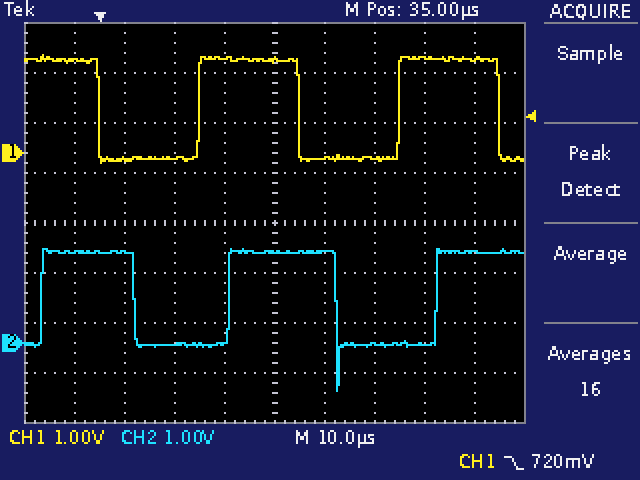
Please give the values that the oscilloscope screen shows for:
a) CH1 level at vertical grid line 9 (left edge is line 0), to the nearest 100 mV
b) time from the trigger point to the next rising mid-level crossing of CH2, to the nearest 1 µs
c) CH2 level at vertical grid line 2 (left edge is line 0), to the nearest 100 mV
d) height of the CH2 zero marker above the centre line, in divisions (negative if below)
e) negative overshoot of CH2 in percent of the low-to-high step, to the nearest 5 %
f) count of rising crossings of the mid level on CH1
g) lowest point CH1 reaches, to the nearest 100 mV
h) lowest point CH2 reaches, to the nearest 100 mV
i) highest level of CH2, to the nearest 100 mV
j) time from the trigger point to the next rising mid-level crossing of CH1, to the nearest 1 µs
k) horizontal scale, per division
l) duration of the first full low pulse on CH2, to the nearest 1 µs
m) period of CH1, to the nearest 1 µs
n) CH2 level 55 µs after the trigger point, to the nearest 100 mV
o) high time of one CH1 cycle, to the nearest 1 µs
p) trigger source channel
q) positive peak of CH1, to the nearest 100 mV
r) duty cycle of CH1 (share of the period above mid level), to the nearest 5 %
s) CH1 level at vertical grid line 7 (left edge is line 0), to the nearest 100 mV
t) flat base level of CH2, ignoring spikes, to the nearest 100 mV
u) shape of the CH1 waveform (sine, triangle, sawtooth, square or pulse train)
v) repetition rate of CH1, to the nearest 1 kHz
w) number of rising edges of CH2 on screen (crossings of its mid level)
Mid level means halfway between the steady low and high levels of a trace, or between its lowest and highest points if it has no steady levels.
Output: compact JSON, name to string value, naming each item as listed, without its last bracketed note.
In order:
{"CH1 level at vertical grid line 9 (left edge is line 0), to the nearest 100 mV": "1.9 V", "time from the trigger point to the next rising mid-level crossing of CH2, to the nearest 1 µs": "26 µs", "CH2 level at vertical grid line 2 (left edge is line 0), to the nearest 100 mV": "1.8 V", "height of the CH2 zero marker above the centre line, in divisions": "-2.4 div", "negative overshoot of CH2 in percent of the low-to-high step, to the nearest 5 %": "50 %", "count of rising crossings of the mid level on CH1": "2", "lowest point CH1 reaches, to the nearest 100 mV": "-200 mV", "lowest point CH2 reaches, to the nearest 100 mV": "-1.0 V", "highest level of CH2, to the nearest 100 mV": "1.9 V", "time from the trigger point to the next rising mid-level crossing of CH1, to the nearest 1 µs": "20 µs", "horizontal scale, per division": "10 µs", "duration of the first full low pulse on CH2, to the nearest 1 µs": "19 µs", "period of CH1, to the nearest 1 µs": "40 µs", "CH2 level 55 µs after the trigger point, to the nearest 100 mV": "0.0 V", "high time of one CH1 cycle, to the nearest 1 µs": "20 µs", "trigger source channel": "CH1", "positive peak of CH1, to the nearest 100 mV": "2.0 V", "duty cycle of CH1 (share of the period above mid level), to the nearest 5 %": "50 %", "CH1 level at vertical grid line 7 (left edge is line 0), to the nearest 100 mV": "-100 mV", "flat base level of CH2, ignoring spikes, to the nearest 100 mV": "0.0 V", "shape of the CH1 waveform": "square", "repetition rate of CH1, to the nearest 1 kHz": "25 kHz", "number of rising edges of CH2 on screen": "3"}
